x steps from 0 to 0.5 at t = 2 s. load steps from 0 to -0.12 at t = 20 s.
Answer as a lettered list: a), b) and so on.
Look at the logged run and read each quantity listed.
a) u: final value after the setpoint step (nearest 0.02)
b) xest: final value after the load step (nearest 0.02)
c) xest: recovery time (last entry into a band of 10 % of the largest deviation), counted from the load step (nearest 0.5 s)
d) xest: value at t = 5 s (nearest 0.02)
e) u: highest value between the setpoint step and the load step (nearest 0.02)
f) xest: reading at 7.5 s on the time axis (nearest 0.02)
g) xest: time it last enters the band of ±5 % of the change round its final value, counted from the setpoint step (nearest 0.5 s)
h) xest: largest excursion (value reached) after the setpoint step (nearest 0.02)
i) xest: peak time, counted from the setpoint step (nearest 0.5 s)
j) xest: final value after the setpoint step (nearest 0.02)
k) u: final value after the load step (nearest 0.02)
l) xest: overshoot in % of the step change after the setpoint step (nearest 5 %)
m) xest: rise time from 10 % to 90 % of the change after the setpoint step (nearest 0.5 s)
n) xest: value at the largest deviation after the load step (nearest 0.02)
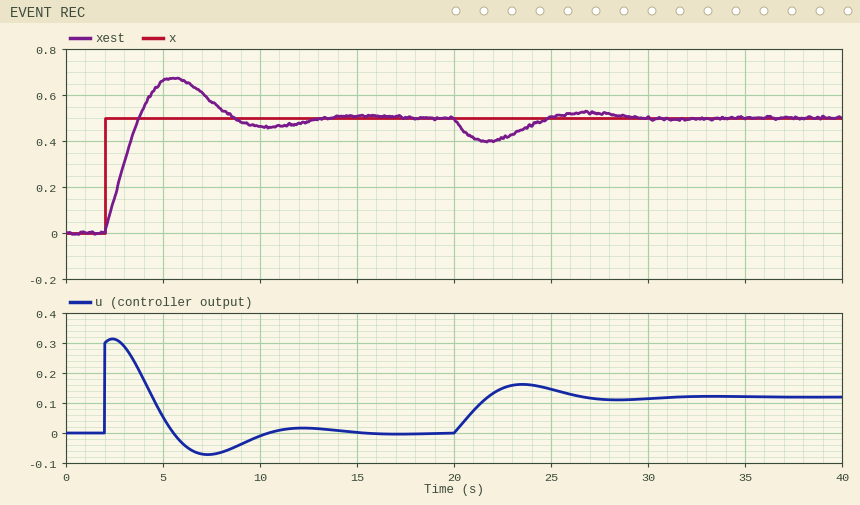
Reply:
a) 0.00
b) 0.50
c) 8.5 s
d) 0.66
e) 0.32
f) 0.58
g) 10.0 s
h) 0.68
i) 3.5 s
j) 0.50
k) 0.12
l) 35 %
m) 1.5 s
n) 0.40
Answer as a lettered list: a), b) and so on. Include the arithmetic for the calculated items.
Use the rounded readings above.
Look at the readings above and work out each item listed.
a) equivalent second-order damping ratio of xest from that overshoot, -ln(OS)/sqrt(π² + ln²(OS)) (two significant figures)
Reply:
a) ln(0.35) = -1.050; 1.050 / sqrt(9.870 + 1.102) = 0.32
